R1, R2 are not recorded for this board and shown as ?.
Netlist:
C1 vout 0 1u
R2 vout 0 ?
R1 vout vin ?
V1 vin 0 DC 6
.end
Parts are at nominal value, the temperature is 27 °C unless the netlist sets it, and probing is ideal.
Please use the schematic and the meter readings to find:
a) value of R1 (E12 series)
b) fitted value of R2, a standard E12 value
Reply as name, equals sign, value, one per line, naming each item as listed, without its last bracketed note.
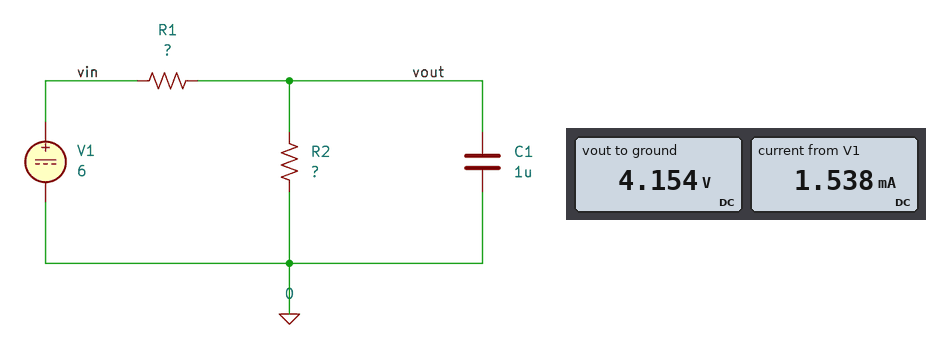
value of R1 = 1.2 kΩ
fitted value of R2, a standard E12 value = 2.7 kΩ
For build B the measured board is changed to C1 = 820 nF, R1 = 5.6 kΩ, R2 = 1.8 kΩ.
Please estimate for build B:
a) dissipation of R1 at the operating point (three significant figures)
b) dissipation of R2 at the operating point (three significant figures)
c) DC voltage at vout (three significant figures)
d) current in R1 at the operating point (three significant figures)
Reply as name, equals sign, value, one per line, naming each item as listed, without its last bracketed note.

dissipation of R1 at the operating point = 3.68 mW
dissipation of R2 at the operating point = 1.18 mW
DC voltage at vout = 1.46 V
current in R1 at the operating point = 811 µA
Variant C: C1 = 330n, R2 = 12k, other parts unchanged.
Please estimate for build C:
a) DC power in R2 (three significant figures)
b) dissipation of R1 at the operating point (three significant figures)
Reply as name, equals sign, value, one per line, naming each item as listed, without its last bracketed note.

DC power in R2 = 2.48 mW
dissipation of R1 at the operating point = 248 µW
